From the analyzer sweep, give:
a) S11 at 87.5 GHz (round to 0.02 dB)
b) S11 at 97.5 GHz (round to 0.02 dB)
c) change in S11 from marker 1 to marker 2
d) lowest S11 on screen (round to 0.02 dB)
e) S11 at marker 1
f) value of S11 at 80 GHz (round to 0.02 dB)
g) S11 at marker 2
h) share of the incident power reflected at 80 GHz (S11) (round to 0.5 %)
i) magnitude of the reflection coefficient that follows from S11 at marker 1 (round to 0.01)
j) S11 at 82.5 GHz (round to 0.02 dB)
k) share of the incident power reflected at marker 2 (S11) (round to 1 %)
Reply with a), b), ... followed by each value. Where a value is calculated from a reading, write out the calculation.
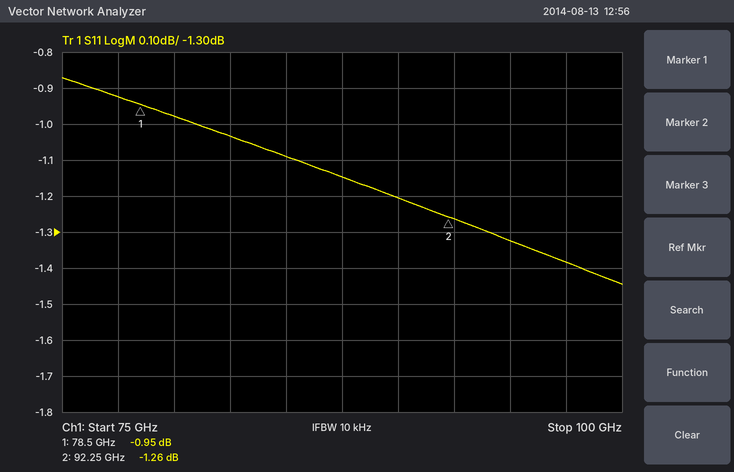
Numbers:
a) -1.14 dB
b) -1.38 dB
c) -1.26 − (-0.95) = -0.31 dB
d) -1.44 dB
e) -0.95 dB
f) -0.98 dB
g) -1.26 dB
h) 10^(-0.98/10) ≈ 79.8 %, so 80.0 % to the nearest 0.5 %
i) 10^(-0.95/20) ≈ 0.90
j) -1.04 dB
k) 10^(-1.26/10) ≈ 75 %
